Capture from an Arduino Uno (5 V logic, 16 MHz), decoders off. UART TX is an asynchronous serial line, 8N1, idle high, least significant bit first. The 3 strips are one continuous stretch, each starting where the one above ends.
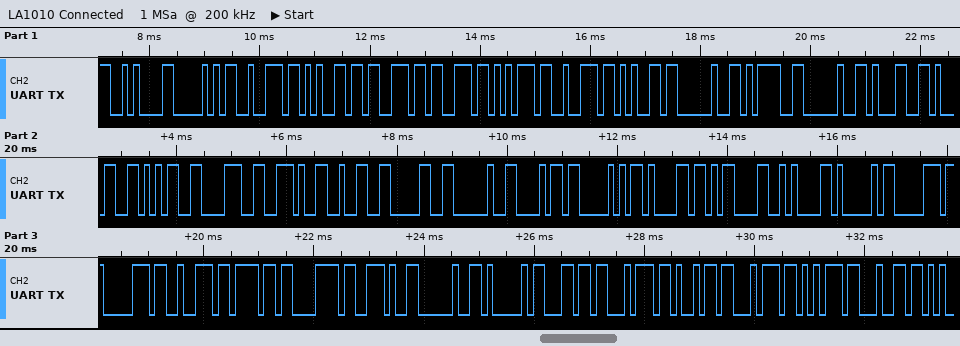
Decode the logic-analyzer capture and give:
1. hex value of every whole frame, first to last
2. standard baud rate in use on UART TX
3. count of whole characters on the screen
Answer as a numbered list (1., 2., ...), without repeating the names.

1. 0A 50 72 65 73 73 75 72 65 20 3D 20 31 31 35 38 2E 32 30 20 68 50 61 0D 0A 41 70 70 72 6F 78 2E 20 41 6C 74 69 74 75 64
2. 9600 baud
3. 40
